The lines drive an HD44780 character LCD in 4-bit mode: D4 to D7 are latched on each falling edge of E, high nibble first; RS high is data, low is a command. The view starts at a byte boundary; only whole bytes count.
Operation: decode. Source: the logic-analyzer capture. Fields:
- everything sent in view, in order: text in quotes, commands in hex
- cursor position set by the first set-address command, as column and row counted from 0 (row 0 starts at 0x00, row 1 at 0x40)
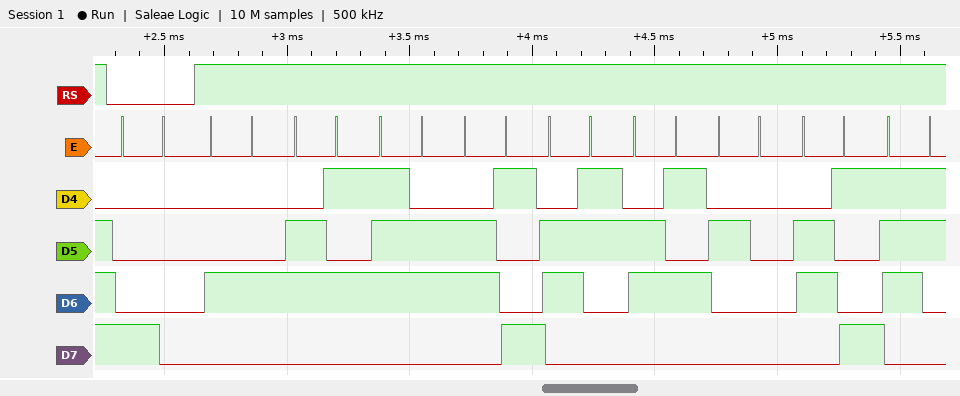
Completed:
0x80 "Device is"
column 0, row 0
